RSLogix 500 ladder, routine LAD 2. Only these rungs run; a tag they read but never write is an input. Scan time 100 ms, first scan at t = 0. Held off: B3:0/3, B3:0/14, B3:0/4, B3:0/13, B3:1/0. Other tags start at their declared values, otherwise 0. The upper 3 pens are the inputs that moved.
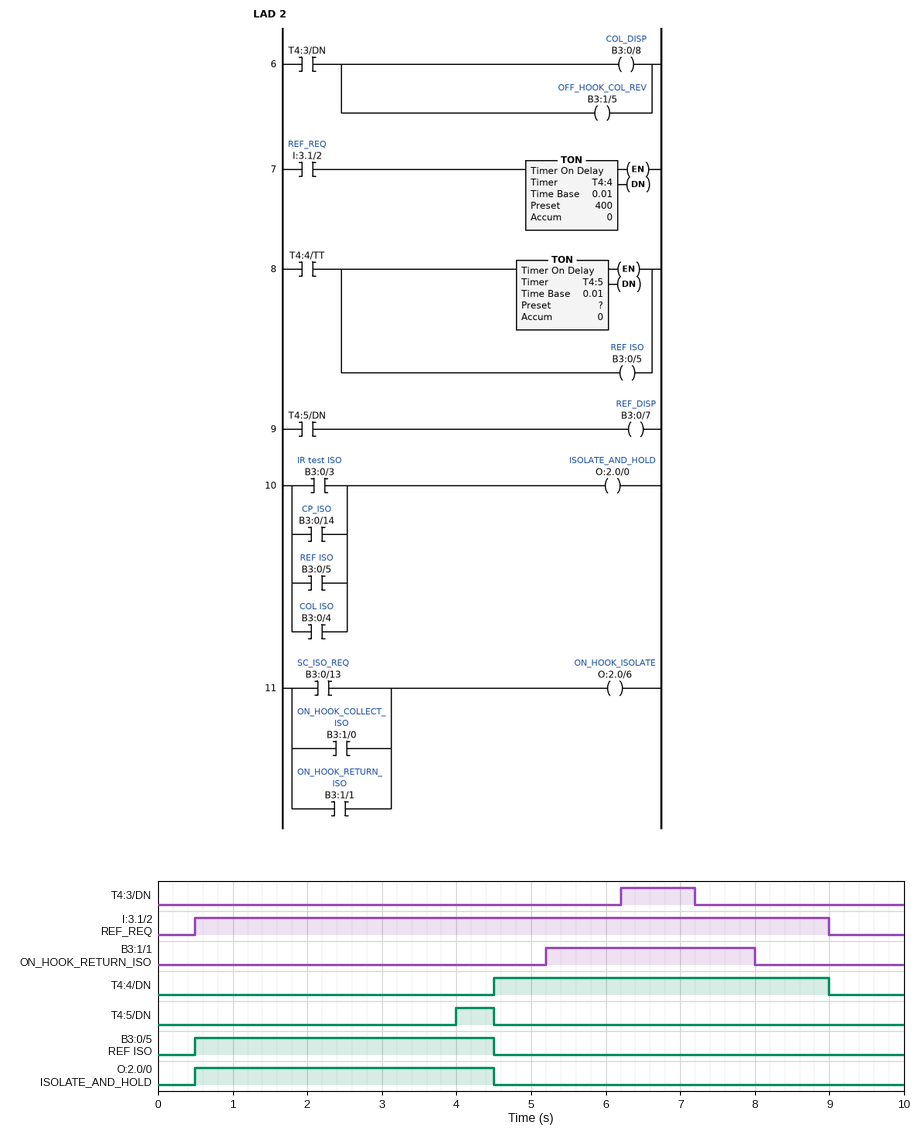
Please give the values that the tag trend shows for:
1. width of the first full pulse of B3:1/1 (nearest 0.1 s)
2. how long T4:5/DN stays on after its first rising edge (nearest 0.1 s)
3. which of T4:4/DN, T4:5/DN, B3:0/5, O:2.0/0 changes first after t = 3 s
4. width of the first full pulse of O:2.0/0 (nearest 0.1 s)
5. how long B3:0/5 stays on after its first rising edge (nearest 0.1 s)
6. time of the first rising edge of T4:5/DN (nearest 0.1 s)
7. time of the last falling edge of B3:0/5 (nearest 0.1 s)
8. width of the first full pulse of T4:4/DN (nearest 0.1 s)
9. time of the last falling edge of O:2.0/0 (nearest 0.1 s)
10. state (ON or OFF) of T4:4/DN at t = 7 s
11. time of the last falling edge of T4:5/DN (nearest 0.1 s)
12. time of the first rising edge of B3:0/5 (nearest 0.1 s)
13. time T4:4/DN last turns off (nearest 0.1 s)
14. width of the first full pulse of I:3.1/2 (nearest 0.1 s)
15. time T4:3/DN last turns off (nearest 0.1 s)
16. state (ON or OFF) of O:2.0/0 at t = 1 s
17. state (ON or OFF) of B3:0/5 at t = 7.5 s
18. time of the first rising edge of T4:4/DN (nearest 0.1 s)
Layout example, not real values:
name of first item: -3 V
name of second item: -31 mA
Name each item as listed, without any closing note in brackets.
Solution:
width of the first full pulse of B3:1/1: 2.8 s
how long T4:5/DN stays on after its first rising edge: 0.5 s
which of T4:4/DN, T4:5/DN, B3:0/5, O:2.0/0 changes first after t = 3 s: T4:5/DN
width of the first full pulse of O:2.0/0: 4.0 s
how long B3:0/5 stays on after its first rising edge: 4.0 s
time of the first rising edge of T4:5/DN: 4.0 s
time of the last falling edge of B3:0/5: 4.5 s
width of the first full pulse of T4:4/DN: 4.5 s
time of the last falling edge of O:2.0/0: 4.5 s
state (ON or OFF) of T4:4/DN at t = 7 s: ON
time of the last falling edge of T4:5/DN: 4.5 s
time of the first rising edge of B3:0/5: 0.5 s
time T4:4/DN last turns off: 9.0 s
width of the first full pulse of I:3.1/2: 8.5 s
time T4:3/DN last turns off: 7.2 s
state (ON or OFF) of O:2.0/0 at t = 1 s: ON
state (ON or OFF) of B3:0/5 at t = 7.5 s: OFF
time of the first rising edge of T4:4/DN: 4.5 s
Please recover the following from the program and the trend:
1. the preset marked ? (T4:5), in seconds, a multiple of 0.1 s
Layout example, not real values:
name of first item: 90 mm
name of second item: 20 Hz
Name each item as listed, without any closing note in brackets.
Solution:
the preset marked ? (T4:5), in seconds, a multiple of 0.1 s: 3.5 s
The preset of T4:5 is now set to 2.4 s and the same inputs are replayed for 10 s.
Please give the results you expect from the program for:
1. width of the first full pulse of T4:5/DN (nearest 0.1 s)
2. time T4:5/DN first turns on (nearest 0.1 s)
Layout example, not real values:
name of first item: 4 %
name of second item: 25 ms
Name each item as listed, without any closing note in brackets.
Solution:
width of the first full pulse of T4:5/DN: 1.6 s
time T4:5/DN first turns on: 2.9 s
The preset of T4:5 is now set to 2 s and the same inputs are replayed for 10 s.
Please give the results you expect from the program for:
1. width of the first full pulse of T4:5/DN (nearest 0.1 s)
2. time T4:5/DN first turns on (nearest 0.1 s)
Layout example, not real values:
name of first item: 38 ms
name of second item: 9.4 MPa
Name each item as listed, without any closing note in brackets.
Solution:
width of the first full pulse of T4:5/DN: 2.0 s
time T4:5/DN first turns on: 2.5 s
